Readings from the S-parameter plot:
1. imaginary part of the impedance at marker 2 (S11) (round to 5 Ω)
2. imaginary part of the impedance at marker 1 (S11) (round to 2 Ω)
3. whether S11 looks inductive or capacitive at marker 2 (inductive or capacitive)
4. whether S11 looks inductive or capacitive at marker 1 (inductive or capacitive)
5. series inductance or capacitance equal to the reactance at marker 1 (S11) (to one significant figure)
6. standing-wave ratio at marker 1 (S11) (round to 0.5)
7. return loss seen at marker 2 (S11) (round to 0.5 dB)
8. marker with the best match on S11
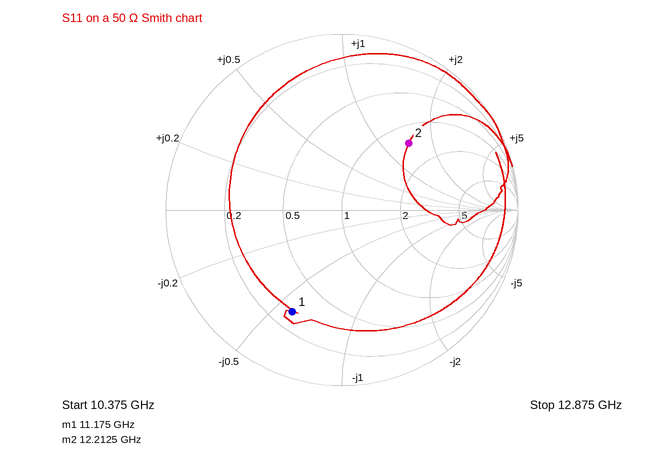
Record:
+70 Ω
-30 Ω
inductive
capacitive
500 fF
4.5
5.5 dB
marker 2
